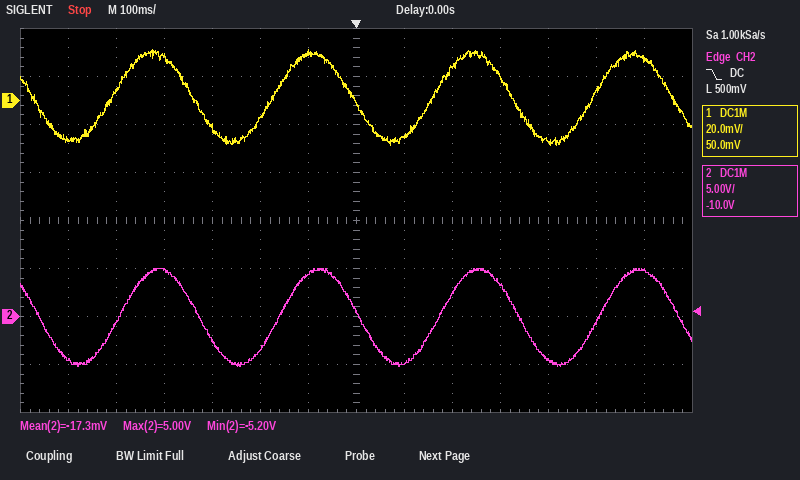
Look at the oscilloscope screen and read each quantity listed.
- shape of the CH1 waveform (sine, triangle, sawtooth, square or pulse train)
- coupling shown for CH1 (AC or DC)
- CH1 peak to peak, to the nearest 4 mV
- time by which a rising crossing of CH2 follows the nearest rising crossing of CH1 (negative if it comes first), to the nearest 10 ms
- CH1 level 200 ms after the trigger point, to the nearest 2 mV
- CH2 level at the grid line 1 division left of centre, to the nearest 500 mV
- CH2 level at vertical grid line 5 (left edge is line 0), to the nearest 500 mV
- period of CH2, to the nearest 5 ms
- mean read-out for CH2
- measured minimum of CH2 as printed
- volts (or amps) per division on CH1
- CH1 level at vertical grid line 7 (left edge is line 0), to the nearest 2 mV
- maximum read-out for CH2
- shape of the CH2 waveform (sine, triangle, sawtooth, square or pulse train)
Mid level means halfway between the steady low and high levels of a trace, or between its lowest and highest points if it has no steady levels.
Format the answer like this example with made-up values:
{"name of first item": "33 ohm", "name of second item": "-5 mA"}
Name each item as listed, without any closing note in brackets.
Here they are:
{"shape of the CH1 waveform": "sine", "coupling shown for CH1": "DC", "CH1 peak to peak, to the nearest 4 mV": "40 mV", "time by which a rising crossing of CH2 follows the nearest rising crossing of CH1 (negative if it comes first), to the nearest 10 ms": "+10 ms", "CH1 level 200 ms after the trigger point, to the nearest 2 mV": "14 mV", "CH2 level at the grid line 1 division left of centre, to the nearest 500 mV": "4.5 V", "CH2 level at vertical grid line 5 (left edge is line 0), to the nearest 500 mV": "-3.5 V", "period of CH2, to the nearest 5 ms": "335 ms", "mean read-out for CH2": "-17.3 mV", "measured minimum of CH2 as printed": "-5.20 V", "volts (or amps) per division on CH1": "20 mV", "CH1 level at vertical grid line 7 (left edge is line 0), to the nearest 2 mV": "0 mV", "maximum read-out for CH2": "5.00 V", "shape of the CH2 waveform": "sine"}
